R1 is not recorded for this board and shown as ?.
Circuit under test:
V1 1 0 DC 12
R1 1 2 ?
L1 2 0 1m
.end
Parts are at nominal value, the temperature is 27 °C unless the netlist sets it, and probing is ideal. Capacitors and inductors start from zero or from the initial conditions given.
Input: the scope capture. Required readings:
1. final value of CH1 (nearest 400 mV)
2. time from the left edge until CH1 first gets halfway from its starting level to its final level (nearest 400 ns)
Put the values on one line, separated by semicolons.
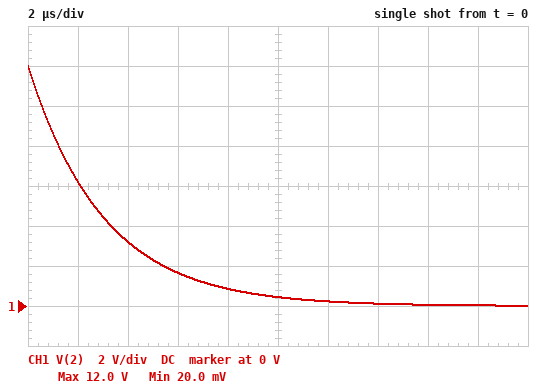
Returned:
0 V; 2.0 µs
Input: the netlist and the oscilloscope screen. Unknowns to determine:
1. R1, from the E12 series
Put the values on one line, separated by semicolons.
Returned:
330 Ω
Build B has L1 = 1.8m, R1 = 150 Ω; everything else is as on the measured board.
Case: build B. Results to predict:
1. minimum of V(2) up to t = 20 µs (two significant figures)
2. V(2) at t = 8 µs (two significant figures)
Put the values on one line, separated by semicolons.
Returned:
2.3 V; 6.2 V
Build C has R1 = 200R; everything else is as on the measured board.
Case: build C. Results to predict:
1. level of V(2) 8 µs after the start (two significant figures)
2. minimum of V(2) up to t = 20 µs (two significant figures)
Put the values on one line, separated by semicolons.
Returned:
2.4 V; 220 mV
